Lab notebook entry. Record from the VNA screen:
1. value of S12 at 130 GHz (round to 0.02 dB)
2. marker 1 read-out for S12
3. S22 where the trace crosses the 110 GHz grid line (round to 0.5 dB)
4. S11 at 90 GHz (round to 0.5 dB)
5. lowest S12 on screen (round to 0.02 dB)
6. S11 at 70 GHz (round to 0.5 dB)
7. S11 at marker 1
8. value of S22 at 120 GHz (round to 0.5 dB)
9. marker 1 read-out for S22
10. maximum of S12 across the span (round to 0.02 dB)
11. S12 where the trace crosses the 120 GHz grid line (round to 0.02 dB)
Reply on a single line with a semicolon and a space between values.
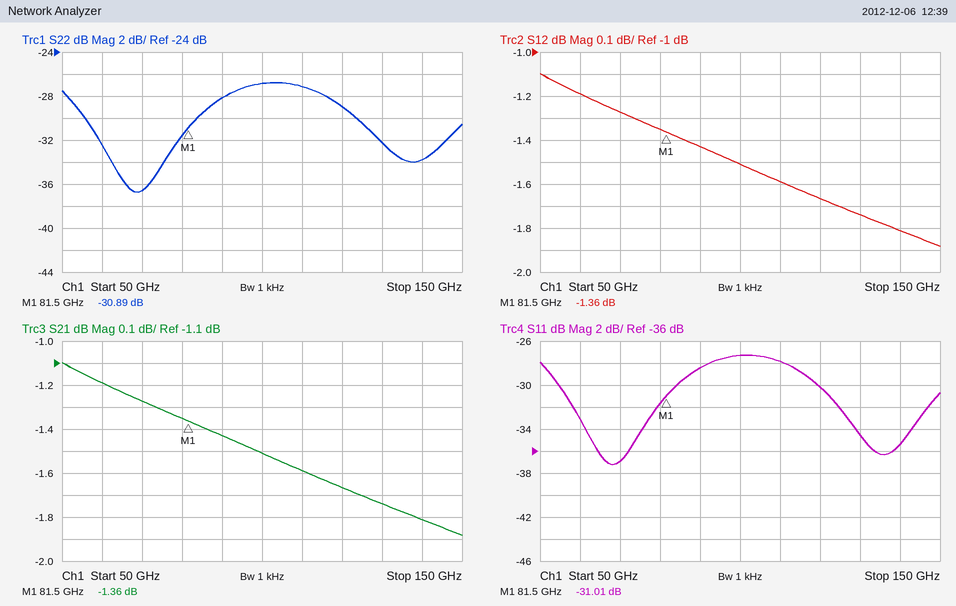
-1.74 dB; -1.36 dB; -27.0 dB; -28.5 dB; -1.88 dB; -37.0 dB; -31.01 dB; -29.0 dB; -30.89 dB; -1.10 dB; -1.66 dB
